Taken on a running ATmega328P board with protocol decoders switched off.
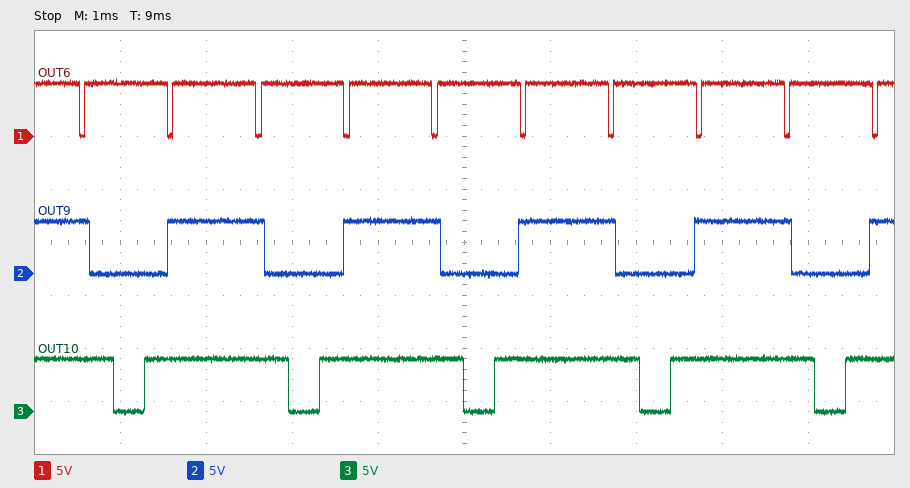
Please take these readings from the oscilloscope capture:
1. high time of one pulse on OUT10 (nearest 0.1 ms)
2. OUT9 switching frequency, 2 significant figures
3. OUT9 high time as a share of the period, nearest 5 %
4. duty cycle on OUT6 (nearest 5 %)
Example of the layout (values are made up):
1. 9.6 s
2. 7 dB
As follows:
1. 1.7 ms
2. 490 Hz
3. 55 %
4. 95 %
